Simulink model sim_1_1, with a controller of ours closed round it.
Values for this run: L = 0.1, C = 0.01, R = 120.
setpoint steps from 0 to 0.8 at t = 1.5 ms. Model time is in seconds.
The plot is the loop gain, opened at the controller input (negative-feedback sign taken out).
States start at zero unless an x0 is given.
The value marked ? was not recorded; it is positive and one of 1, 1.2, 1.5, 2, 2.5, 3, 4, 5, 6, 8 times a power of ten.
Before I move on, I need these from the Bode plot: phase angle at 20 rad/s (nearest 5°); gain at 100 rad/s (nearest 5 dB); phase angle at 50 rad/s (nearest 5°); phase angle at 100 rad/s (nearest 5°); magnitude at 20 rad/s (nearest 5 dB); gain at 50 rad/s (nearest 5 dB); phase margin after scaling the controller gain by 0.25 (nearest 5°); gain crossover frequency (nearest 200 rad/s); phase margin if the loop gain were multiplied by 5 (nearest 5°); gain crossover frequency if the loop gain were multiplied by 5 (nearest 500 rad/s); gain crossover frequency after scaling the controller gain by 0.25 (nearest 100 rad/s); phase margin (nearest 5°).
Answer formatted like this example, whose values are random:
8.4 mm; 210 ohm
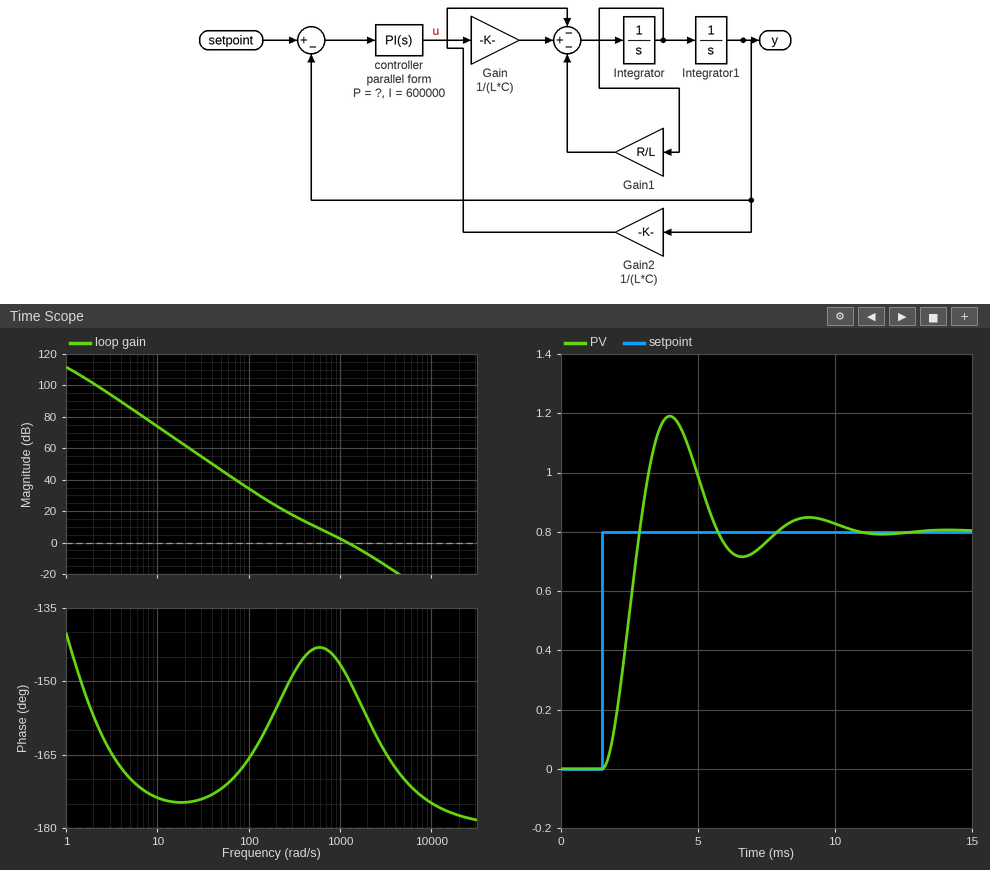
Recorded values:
-175°; 35 dB; -170°; -165°; 60 dB; 45 dB; 35°; 1200 rad/s; 15°; 3000 rad/s; 500 rad/s; 30°
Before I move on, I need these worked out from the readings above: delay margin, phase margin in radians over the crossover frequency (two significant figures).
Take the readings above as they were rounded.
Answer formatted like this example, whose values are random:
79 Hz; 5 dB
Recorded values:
0.00044 s
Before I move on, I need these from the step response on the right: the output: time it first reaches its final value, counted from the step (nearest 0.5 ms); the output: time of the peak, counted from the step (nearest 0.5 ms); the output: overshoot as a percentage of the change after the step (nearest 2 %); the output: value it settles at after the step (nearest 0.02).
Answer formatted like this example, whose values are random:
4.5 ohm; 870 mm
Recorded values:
1.5 ms; 2.5 ms; 48 %; 0.80
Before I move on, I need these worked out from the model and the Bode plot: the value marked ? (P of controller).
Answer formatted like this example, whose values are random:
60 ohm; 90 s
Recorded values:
2000
